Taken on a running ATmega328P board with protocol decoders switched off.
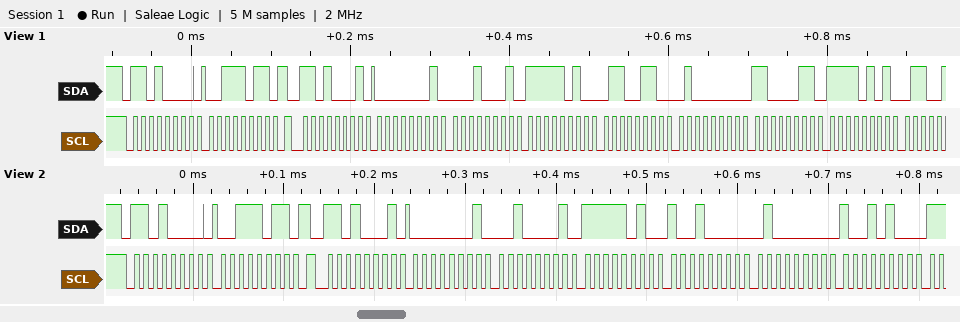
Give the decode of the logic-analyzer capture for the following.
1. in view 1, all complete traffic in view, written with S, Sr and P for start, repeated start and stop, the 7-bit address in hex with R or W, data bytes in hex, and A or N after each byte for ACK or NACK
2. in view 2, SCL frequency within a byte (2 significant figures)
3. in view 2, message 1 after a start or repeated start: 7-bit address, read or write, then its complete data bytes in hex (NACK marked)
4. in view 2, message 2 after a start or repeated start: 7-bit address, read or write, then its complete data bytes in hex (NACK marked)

S 68W A 3B A Sr 68R A 01 A 11 A FA A 66 A 40 A C3 A F5 A
100 kHz
0x68 write: 3B
0x68 read: 01 21 FA 90 40 94
